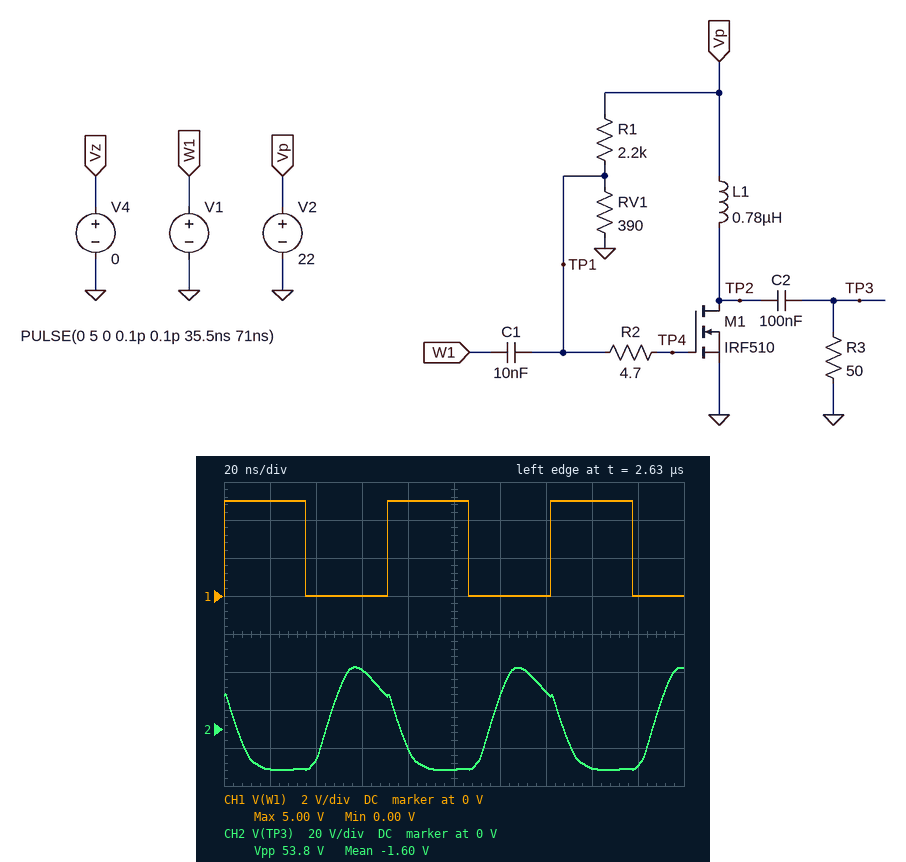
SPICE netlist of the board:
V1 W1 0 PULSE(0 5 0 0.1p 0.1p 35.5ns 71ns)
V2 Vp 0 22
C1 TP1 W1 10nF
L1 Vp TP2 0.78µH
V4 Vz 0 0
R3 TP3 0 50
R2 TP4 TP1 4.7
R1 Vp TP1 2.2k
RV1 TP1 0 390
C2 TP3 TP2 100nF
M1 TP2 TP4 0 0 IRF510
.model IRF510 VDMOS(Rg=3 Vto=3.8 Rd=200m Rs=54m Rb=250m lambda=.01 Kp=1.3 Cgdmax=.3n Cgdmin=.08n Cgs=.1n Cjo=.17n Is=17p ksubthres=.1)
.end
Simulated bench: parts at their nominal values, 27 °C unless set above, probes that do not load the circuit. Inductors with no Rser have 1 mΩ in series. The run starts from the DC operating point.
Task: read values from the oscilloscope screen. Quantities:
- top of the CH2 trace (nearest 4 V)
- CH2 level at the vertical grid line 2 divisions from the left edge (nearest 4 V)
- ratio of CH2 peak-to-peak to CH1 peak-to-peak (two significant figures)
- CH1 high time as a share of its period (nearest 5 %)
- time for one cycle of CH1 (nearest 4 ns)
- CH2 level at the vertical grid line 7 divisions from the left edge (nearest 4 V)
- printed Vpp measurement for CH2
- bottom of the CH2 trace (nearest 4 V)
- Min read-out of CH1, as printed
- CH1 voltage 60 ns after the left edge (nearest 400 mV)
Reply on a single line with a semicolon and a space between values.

32 V; -16 V; 11; 50 %; 72 ns; 20 V; 53.8 V; -20 V; 0.00 V; 0 V
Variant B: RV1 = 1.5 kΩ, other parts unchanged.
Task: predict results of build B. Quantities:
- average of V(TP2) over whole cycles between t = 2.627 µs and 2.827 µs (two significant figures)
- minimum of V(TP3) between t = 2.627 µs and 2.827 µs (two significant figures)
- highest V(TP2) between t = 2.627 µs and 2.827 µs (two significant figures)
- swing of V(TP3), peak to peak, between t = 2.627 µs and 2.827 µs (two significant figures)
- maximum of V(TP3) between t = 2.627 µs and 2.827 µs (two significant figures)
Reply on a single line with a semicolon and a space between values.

23 V; -14 V; 57 V; 49 V; 35 V
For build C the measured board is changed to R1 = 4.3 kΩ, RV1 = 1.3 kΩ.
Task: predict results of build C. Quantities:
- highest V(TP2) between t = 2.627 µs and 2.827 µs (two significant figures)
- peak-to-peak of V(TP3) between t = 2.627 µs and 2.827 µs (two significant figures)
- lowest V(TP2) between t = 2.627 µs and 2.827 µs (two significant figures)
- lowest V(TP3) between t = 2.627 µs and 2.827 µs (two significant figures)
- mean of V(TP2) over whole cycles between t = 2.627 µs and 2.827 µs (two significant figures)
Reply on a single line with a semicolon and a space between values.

64 V; 62 V; 1.9 V; -20 V; 22 V
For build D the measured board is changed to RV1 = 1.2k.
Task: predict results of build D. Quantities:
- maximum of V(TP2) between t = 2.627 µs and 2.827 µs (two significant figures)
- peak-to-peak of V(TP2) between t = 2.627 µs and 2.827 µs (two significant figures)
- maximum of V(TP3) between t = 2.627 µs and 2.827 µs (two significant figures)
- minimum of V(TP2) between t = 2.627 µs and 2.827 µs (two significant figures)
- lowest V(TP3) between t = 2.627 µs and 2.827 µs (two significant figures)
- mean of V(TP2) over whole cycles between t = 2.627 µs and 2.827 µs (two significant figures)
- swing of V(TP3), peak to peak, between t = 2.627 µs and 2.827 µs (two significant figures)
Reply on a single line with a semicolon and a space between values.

60 V; 55 V; 38 V; 5.3 V; -16 V; 23 V; 55 V
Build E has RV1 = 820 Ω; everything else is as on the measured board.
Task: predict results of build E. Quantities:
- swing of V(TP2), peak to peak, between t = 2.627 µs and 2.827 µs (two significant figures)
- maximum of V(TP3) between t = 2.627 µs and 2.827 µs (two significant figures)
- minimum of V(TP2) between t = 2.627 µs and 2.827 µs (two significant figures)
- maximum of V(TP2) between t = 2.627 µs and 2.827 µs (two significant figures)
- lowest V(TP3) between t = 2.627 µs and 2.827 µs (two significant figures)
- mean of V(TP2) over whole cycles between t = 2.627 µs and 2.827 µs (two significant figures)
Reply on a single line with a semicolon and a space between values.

61 V; 42 V; 2.6 V; 64 V; -19 V; 23 V
